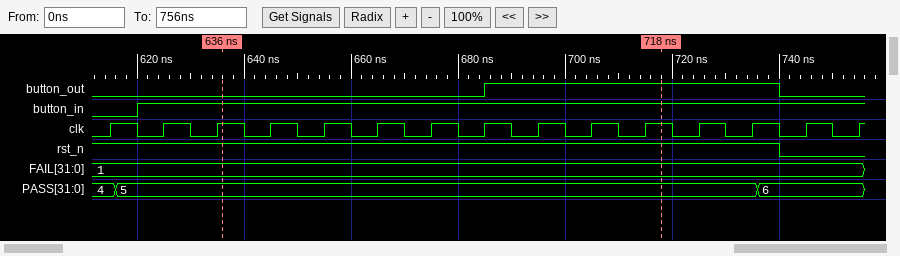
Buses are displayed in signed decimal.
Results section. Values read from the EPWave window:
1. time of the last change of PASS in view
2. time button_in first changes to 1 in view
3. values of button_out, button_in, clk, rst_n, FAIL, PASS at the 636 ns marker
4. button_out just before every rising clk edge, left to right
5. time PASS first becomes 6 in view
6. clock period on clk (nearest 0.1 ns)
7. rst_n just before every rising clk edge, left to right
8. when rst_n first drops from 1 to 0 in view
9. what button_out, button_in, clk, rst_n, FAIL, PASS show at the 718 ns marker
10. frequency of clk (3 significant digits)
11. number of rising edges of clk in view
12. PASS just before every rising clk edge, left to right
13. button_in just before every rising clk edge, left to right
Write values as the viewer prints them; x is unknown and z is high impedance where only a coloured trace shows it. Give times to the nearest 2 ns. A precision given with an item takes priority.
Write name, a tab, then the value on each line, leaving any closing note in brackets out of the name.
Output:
time of the last change of PASS in view	736 ns
time button_in first changes to 1 in view	620 ns
values of button_out, button_in, clk, rst_n, FAIL, PASS at the 636 ns marker	button_out=0, button_in=1, clk=1, rst_n=1, FAIL=1, PASS=5
button_out just before every rising clk edge, left to right	0 0 0 0 0 0 0 0 1 1 1 1 1 0 0
time PASS first becomes 6 in view	736 ns
clock period on clk	10 ns
rst_n just before every rising clk edge, left to right	1 1 1 1 1 1 1 1 1 1 1 1 1 0 0
when rst_n first drops from 1 to 0 in view	740 ns
what button_out, button_in, clk, rst_n, FAIL, PASS show at the 718 ns marker	button_out=1, button_in=1, clk=1, rst_n=1, FAIL=1, PASS=5
frequency of clk	100 MHz
number of rising edges of clk in view	15
PASS just before every rising clk edge, left to right	4, 5, 5, 5, 5, 5, 5, 5, 5, 5, 5, 5, 5, 6, 6
button_in just before every rising clk edge, left to right	0 1 1 1 1 1 1 1 1 1 1 1 1 1 1
